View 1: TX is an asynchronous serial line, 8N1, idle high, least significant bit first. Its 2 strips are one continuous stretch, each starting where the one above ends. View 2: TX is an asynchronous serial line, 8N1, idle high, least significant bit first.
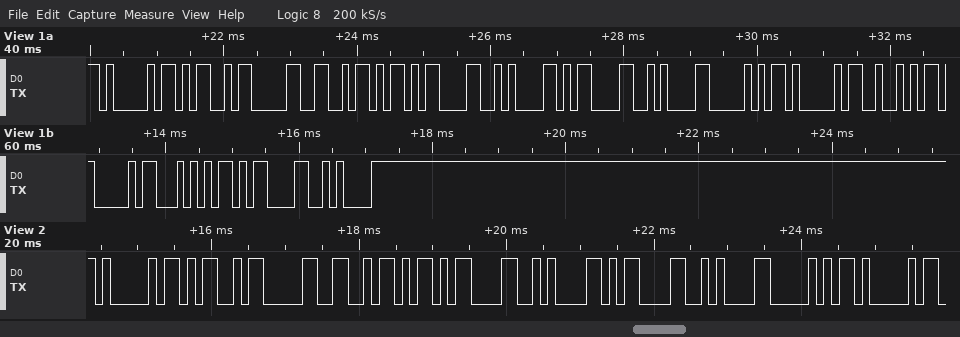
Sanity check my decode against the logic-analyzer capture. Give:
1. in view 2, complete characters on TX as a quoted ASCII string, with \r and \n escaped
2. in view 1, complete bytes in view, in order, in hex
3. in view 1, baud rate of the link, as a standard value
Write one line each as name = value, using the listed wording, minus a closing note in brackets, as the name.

in view 2, complete characters on TX as a quoted ASCII string, with \r and \n escaped = "AM0Z\r\n\r\nPA"
in view 1, complete bytes in view, in order, in hex = 41 4D 30 5A 0D 0A 0D 0A 50 41 52 41 54 0D 0A
in view 1, baud rate of the link, as a standard value = 9600 baud
